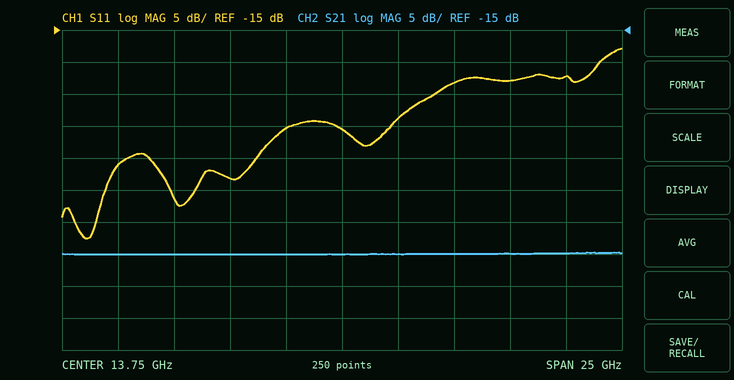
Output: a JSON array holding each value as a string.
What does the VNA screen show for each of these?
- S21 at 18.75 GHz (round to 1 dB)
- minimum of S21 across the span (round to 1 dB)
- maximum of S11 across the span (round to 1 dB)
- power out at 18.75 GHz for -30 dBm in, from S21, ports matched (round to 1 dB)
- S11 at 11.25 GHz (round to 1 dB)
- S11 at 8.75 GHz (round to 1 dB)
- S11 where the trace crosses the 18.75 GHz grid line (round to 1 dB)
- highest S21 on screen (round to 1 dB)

["-50 dB", "-50 dB", "-18 dB", "-80 dBm", "-30 dB", "-38 dB", "-23 dB", "-50 dB"]
